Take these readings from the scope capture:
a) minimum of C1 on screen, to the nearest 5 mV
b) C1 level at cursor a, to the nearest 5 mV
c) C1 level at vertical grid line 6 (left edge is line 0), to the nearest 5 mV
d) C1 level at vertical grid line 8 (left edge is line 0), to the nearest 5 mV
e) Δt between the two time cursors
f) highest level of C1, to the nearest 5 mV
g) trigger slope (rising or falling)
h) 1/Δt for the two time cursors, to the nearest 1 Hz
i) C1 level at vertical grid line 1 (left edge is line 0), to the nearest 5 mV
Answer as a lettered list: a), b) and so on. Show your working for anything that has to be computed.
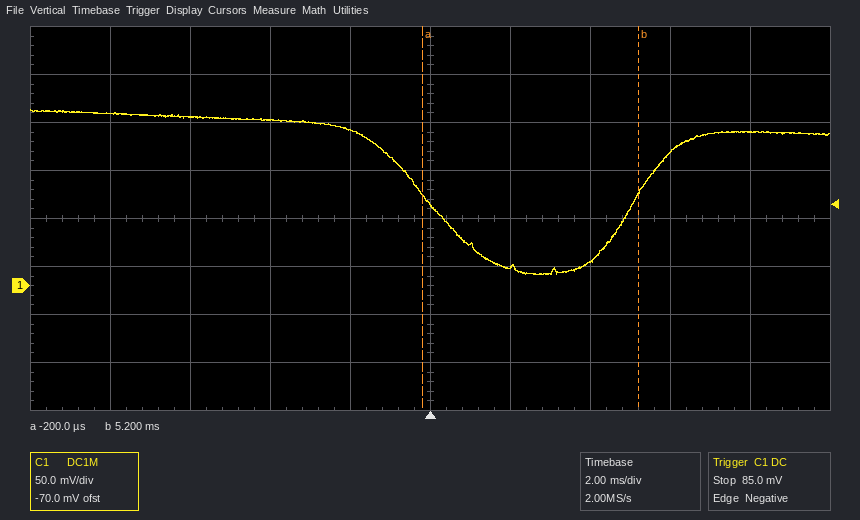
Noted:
a) 10 mV
b) 95 mV
c) 20 mV
d) 140 mV
e) 5.2 ms − (-200 µs) = 5.4 ms
f) 185 mV
g) falling
h) 1 / 5.4 ms ≈ 185 Hz
i) 180 mV
